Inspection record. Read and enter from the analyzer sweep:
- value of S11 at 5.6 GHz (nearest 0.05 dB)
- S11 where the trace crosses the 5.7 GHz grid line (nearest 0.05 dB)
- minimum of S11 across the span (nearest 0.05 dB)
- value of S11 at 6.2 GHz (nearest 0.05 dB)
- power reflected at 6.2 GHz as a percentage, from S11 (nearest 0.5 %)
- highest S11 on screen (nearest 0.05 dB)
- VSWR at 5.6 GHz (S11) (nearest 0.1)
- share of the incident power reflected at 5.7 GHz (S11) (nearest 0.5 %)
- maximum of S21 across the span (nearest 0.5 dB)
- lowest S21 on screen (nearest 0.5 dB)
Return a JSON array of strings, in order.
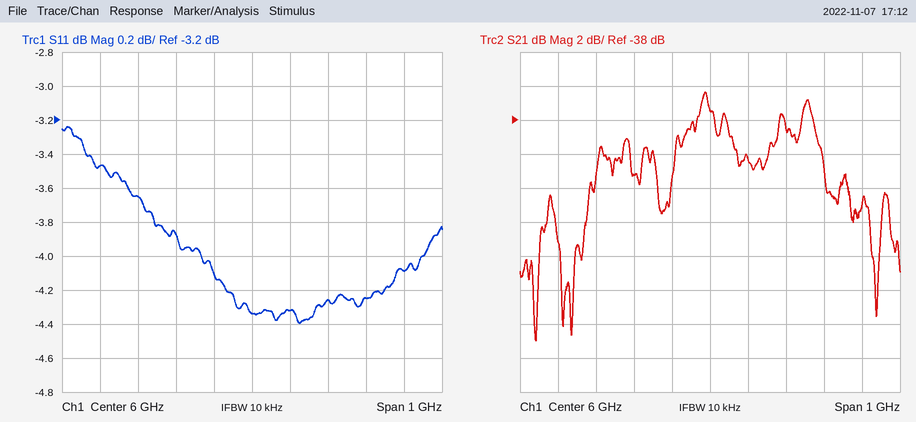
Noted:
["-3.45 dB", "-3.65 dB", "-4.40 dB", "-4.25 dB", "37.5 %", "-3.25 dB", "5.1", "43.0 %", "-36.5 dB", "-51.0 dB"]
